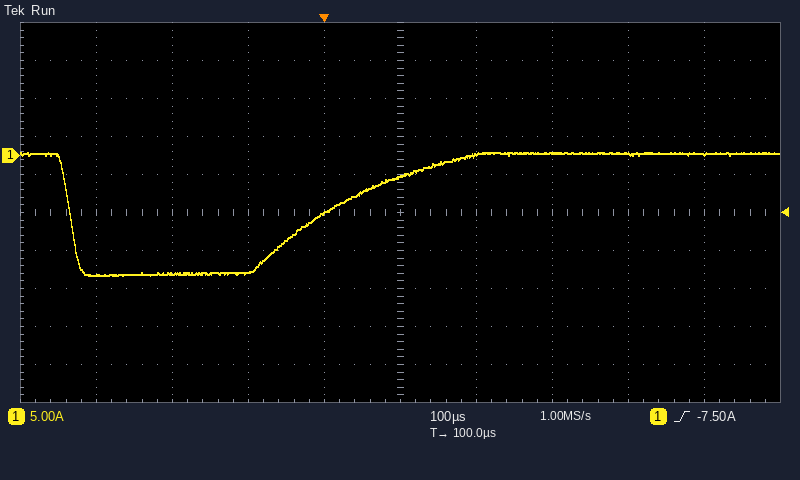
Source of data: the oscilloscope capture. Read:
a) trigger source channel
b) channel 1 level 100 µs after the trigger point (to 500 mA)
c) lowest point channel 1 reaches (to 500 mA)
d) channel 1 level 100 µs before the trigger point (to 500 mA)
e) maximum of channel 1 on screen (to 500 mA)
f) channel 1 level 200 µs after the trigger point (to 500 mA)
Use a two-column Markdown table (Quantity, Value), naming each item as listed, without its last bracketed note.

| Quantity | Value |
|---|---|
| trigger source channel | channel 1 |
| channel 1 level 100 µs after the trigger point | -3.0 A |
| lowest point channel 1 reaches | -16.0 A |
| channel 1 level 100 µs before the trigger point | -15.5 A |
| maximum of channel 1 on screen | 500 mA |
| channel 1 level 200 µs after the trigger point | 0.0 A |
